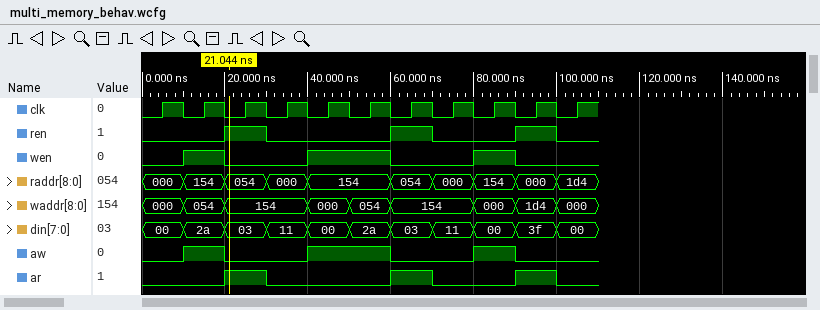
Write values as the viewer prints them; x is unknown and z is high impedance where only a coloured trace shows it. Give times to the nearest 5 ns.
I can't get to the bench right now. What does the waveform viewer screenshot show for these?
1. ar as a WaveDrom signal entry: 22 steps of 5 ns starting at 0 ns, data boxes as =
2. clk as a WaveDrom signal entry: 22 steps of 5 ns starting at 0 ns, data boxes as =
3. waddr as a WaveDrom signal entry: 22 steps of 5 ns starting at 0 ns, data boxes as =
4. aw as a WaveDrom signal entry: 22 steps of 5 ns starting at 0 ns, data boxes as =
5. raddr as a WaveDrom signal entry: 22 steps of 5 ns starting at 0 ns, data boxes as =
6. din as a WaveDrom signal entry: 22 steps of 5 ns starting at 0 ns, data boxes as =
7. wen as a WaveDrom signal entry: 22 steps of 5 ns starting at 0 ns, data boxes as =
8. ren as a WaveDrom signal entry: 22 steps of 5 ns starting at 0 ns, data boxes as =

{name: 'ar', wave: '0...1.0.....1.0...1.0.'}
{name: 'clk', wave: '0101010101010101010101'}
{name: 'waddr', wave: '=.=.=...=.=.=...=.=.=.', data: '000 054 154 000 054 154 000 1d4 000'}
{name: 'aw', wave: '0.1.0...1...0...1.0...'}
{name: 'raddr', wave: '=.=.=.=.=...=.=.=.=.=.', data: '000 154 054 000 154 054 000 154 000 1d4'}
{name: 'din', wave: '=.=.=.=.=.=.=.=.=.=.=.', data: '00 2a 03 11 00 2a 03 11 00 3f 00'}
{name: 'wen', wave: '0.1.0...1...0...1.0...'}
{name: 'ren', wave: '0...1.0.....1.0...1.0.'}
